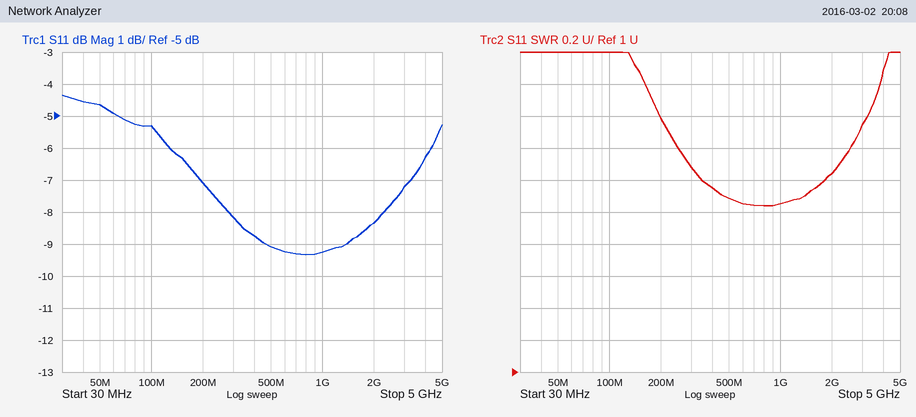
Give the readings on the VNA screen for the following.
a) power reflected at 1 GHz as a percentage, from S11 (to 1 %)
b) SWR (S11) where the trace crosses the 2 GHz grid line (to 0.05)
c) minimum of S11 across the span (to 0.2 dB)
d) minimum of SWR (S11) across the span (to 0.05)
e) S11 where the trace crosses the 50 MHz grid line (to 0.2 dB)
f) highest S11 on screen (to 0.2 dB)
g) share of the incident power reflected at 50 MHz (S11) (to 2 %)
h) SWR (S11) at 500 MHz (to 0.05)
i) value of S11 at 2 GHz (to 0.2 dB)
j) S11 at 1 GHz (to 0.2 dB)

12 %
2.25
-9.4 dB
2.05
-4.6 dB
-4.4 dB
34 %
2.10
-8.4 dB
-9.2 dB
